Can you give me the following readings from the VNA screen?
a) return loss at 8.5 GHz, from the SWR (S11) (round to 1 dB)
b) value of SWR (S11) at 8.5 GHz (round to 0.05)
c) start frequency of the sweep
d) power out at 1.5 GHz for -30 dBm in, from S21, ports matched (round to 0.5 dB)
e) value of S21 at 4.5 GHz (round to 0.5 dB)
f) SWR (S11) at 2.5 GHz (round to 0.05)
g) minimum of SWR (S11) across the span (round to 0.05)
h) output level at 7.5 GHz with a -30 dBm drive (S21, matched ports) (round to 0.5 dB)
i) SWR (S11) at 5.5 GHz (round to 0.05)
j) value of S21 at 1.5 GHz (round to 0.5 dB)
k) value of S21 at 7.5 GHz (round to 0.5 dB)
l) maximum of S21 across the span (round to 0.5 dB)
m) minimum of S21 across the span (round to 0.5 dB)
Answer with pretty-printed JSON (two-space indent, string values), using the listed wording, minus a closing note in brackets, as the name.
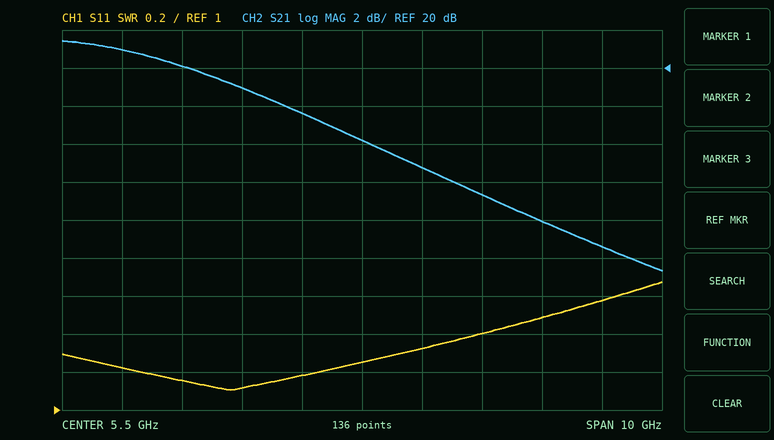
{
  "return loss at 8.5 GHz, from the SWR (S11)": "14 dB",
  "value of SWR (S11) at 8.5 GHz": "1.50",
  "start frequency of the sweep": "500 MHz",
  "power out at 1.5 GHz for -30 dBm in, from S21, ports matched": "-9.0 dBm",
  "value of S21 at 4.5 GHz": "17.5 dB",
  "SWR (S11) at 2.5 GHz": "1.15",
  "minimum of SWR (S11) across the span": "1.10",
  "output level at 7.5 GHz with a -30 dBm drive (S21, matched ports)": "-16.5 dBm",
  "SWR (S11) at 5.5 GHz": "1.25",
  "value of S21 at 1.5 GHz": "21.0 dB",
  "value of S21 at 7.5 GHz": "13.5 dB",
  "maximum of S21 across the span": "21.5 dB",
  "minimum of S21 across the span": "9.5 dB"
}
